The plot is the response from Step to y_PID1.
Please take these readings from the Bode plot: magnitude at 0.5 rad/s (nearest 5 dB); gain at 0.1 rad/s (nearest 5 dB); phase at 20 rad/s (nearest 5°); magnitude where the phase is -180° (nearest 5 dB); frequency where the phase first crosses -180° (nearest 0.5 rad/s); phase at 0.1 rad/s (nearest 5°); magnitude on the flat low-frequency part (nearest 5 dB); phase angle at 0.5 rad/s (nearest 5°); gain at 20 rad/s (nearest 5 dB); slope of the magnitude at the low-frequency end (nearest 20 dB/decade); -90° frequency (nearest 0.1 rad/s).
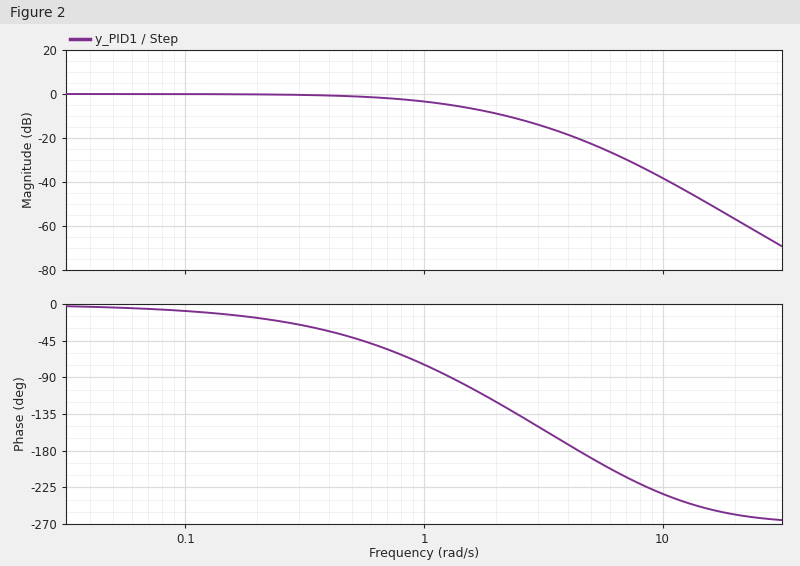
0 dB
0 dB
-260°
-20 dB
4.5 rad/s
-10°
0 dB
-40°
-55 dB
0 dB/decade
1.3 rad/s
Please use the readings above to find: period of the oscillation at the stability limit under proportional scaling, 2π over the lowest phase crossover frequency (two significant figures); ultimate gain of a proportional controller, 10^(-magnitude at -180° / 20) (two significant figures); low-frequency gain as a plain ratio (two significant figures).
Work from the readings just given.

1.4 s
10
1.0
